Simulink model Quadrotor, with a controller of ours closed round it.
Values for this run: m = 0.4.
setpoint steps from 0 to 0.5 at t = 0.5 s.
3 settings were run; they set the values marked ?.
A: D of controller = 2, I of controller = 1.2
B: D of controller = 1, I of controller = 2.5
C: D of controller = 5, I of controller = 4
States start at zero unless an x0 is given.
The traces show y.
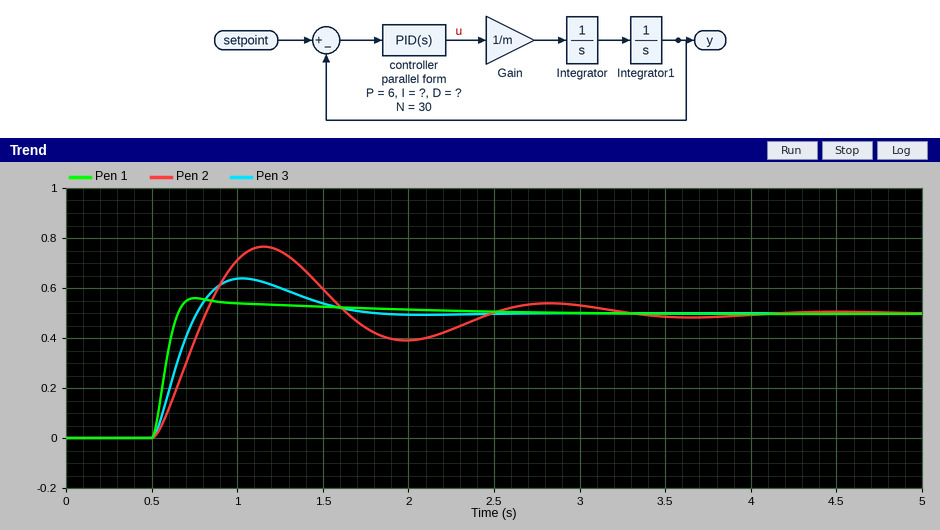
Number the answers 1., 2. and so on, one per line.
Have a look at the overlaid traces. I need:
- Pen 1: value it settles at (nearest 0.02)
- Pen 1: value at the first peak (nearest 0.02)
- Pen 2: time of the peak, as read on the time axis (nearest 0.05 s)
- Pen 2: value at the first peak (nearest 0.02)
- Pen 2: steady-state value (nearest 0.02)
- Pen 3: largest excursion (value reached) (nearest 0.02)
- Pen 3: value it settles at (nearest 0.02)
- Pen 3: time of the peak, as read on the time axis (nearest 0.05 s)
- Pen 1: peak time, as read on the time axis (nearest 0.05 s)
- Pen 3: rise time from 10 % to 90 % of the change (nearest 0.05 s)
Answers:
1. 0.50
2. 0.56
3. 1.15 s
4. 0.76
5. 0.50
6. 0.64
7. 0.50
8. 1.05 s
9. 0.75 s
10. 0.20 s
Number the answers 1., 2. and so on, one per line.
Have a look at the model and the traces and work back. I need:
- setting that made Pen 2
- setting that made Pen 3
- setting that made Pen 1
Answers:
1. B
2. A
3. C
